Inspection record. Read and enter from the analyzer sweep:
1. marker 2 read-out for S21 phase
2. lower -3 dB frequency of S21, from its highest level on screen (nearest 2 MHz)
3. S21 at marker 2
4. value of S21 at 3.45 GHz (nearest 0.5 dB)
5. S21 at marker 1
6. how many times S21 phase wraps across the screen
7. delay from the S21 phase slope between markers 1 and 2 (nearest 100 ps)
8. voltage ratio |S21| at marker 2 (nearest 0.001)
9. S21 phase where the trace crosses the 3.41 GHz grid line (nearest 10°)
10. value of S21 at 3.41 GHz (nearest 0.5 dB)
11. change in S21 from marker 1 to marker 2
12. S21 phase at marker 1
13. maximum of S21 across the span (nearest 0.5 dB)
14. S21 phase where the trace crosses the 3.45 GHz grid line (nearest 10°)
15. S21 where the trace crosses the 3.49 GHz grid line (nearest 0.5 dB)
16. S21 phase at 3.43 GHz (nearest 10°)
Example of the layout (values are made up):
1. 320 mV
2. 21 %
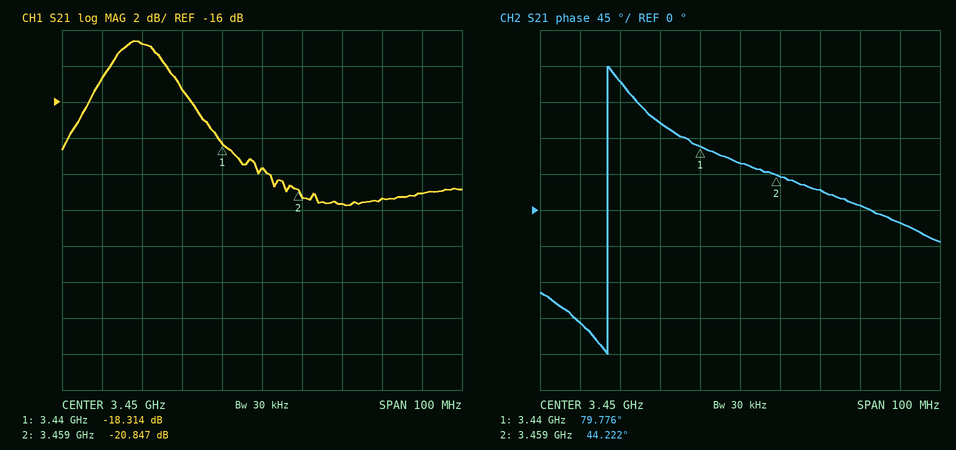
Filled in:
1. 44.222°
2. 3.408 GHz
3. -20.847 dB
4. -19.5 dB
5. -18.314 dB
6. 1
7. 5.2 ns
8. 0.091
9. -140°
10. -14.5 dB
11. -2.533 dB
12. 79.776°
13. -12.5 dB
14. 60°
15. -21.0 dB
16. 110°
